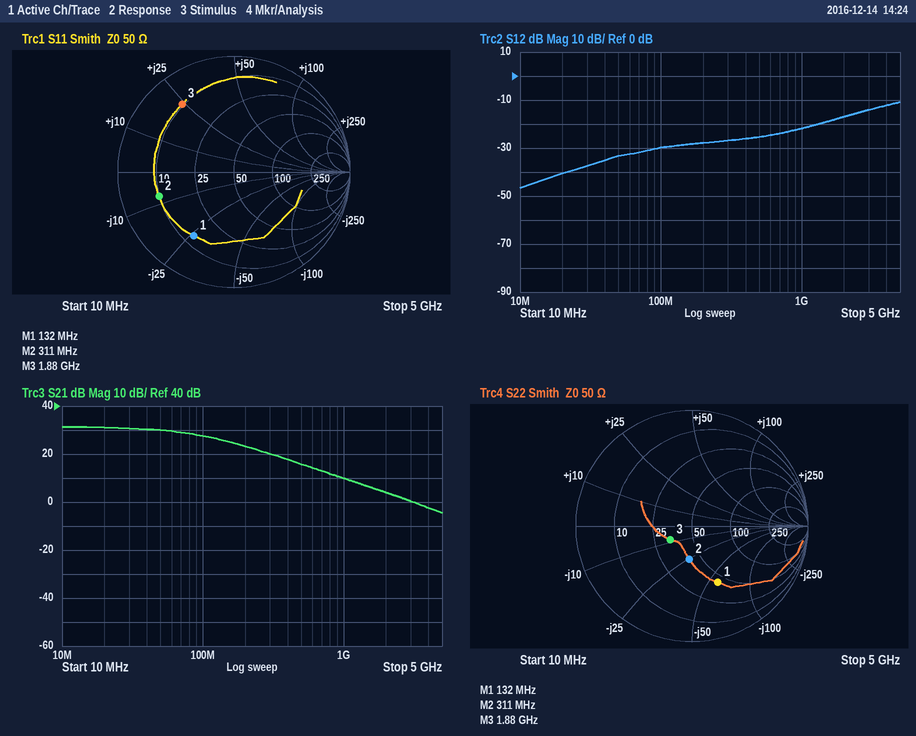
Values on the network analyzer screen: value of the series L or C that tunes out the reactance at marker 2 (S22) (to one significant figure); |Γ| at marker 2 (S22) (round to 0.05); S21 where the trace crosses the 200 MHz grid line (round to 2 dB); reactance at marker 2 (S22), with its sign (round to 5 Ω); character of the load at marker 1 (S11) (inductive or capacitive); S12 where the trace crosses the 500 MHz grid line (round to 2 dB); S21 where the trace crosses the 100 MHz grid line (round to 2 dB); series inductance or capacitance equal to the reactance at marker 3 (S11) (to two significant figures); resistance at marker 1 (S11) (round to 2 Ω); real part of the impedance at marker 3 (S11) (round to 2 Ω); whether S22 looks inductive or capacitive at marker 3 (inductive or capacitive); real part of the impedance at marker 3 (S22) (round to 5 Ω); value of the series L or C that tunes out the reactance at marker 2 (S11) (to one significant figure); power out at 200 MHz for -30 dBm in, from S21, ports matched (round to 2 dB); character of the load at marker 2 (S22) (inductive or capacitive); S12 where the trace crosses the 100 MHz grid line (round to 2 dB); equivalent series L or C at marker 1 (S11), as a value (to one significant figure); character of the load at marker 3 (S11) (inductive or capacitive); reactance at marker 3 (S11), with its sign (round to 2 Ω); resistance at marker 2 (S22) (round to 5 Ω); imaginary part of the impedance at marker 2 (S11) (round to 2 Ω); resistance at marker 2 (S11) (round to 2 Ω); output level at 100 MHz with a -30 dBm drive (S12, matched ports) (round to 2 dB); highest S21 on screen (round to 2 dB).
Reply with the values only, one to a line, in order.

10 nH
0.30
24 dB
-25 Ω
capacitive
-26 dB
28 dB
2.0 nH
14 Ω
10 Ω
capacitive
35 Ω
4 nH
-6 dBm
capacitive
-30 dB
50 pF
inductive
+24 Ω
40 Ω
-8 Ω
10 Ω
-60 dBm
32 dB
